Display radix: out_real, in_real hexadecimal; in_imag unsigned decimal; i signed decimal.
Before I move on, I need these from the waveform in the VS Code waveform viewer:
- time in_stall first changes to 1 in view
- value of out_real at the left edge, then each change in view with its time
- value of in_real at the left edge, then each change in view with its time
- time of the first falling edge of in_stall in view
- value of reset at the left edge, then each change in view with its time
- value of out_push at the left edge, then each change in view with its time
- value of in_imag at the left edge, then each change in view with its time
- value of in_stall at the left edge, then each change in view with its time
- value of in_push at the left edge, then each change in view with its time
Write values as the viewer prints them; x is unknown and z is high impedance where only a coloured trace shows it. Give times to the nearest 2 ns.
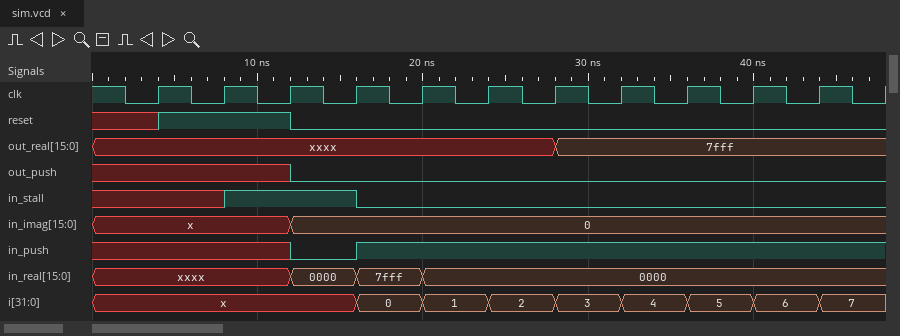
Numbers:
8 ns
xxxx, 7fff at 28 ns
xxxx, 0000 at 12 ns, 7fff at 16 ns, 0000 at 20 ns
16 ns
x, 1 at 4 ns, 0 at 12 ns
x, 0 at 12 ns
x, 0 at 12 ns
x, 1 at 8 ns, 0 at 16 ns
x, 0 at 12 ns, 1 at 16 ns
